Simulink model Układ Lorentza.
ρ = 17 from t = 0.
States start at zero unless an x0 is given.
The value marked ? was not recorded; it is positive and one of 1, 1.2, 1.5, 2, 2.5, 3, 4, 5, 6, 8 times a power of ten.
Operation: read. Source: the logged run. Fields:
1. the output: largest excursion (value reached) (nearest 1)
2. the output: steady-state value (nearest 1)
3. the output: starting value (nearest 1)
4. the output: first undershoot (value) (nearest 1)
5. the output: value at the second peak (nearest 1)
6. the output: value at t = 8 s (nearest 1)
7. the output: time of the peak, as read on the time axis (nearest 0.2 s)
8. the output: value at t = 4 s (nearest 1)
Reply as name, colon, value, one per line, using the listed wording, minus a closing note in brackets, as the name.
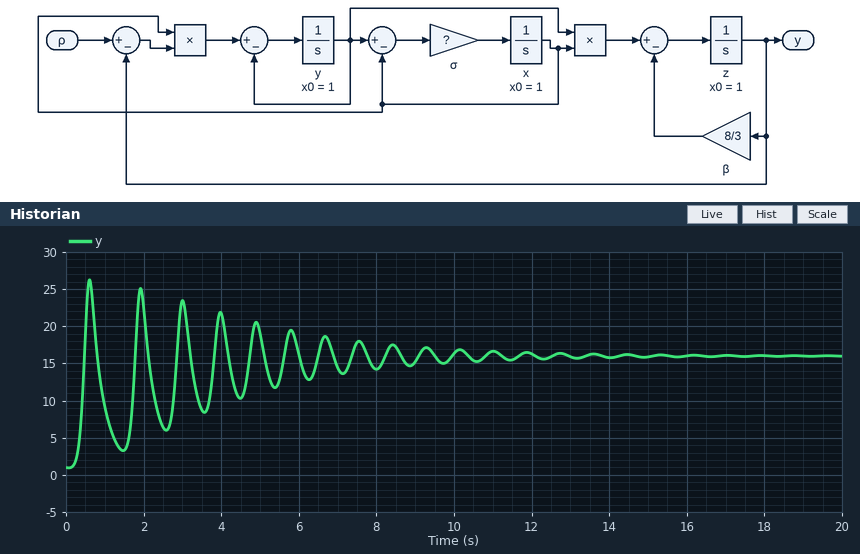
the output: largest excursion (value reached): 26
the output: steady-state value: 16
the output: starting value: 1
the output: first undershoot (value): 3
the output: value at the second peak: 25
the output: value at t = 8 s: 14
the output: time of the peak, as read on the time axis: 0.6 s
the output: value at t = 4 s: 22
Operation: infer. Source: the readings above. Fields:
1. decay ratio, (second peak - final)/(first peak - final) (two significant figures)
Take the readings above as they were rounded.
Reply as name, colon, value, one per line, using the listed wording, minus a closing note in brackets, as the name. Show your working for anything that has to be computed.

decay ratio, (second peak - final)/(first peak - final): (25 - 16) / (26 - 16) = 0.90
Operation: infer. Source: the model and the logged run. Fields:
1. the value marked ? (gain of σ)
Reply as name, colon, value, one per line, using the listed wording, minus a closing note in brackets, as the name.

the value marked ?: 5
